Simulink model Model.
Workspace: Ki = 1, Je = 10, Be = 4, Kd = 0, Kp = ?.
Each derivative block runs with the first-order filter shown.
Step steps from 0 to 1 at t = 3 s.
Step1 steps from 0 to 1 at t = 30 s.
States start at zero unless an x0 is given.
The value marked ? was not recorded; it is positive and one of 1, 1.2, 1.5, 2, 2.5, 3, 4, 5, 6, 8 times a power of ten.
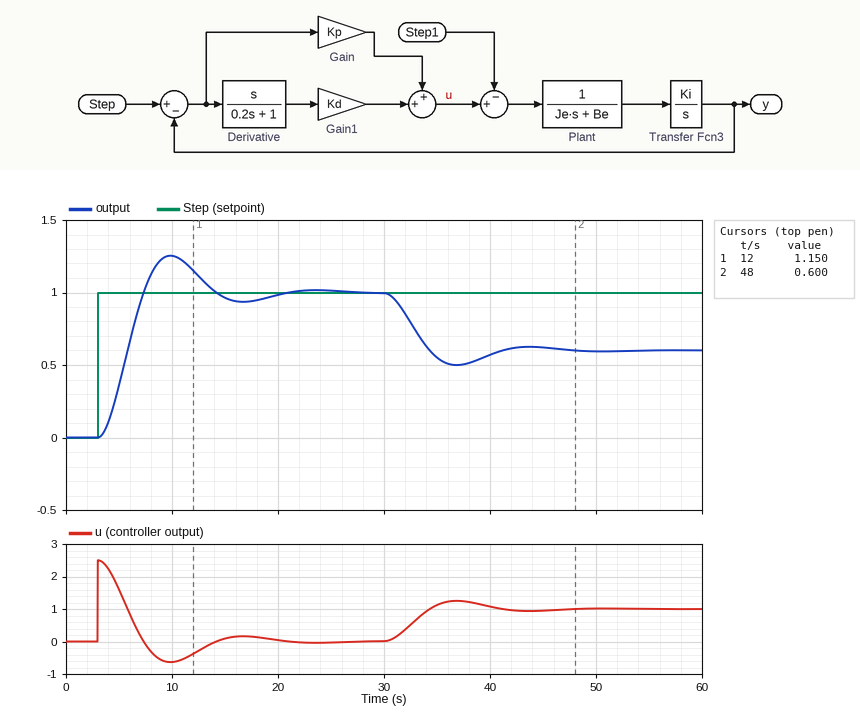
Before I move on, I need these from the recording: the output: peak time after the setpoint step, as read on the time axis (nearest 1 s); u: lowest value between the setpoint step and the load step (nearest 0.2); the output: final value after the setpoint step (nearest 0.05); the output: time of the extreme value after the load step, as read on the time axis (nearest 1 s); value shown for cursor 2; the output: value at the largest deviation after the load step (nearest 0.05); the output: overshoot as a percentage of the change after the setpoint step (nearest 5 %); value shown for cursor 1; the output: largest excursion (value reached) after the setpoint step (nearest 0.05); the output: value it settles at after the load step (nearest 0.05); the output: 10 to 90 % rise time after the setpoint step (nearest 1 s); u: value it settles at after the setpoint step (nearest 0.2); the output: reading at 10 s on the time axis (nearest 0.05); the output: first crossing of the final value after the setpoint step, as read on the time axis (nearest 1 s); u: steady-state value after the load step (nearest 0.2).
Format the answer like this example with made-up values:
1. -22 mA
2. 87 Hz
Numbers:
1. 10 s
2. -0.6
3. 1.00
4. 37 s
5. 0.600
6. 0.50
7. 25 %
8. 1.150
9. 1.25
10. 0.60
11. 3 s
12. 0.0
13. 1.25
14. 7 s
15. 1.0
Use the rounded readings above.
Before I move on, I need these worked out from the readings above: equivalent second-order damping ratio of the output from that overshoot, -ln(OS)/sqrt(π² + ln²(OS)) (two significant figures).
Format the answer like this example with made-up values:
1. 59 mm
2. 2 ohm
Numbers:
1. 0.40
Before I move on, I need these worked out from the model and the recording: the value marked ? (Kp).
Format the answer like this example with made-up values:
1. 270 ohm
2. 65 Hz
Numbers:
1. 2.5
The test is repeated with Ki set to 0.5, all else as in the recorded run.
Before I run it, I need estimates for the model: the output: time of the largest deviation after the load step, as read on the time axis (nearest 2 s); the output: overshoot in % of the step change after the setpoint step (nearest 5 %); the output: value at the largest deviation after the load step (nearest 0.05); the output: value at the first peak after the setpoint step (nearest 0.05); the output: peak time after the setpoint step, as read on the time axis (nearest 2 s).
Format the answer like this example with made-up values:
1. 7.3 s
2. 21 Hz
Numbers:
1. 40 s
2. 10 %
3. 0.55
4. 1.10
5. 14 s
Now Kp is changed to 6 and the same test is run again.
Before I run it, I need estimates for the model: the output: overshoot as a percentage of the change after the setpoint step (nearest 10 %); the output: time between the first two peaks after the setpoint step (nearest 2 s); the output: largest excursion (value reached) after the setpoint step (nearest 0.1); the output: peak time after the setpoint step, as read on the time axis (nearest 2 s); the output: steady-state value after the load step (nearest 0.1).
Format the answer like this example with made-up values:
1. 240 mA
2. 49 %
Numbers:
1. 40 %
2. 8 s
3. 1.4
4. 8 s
5. 0.8
